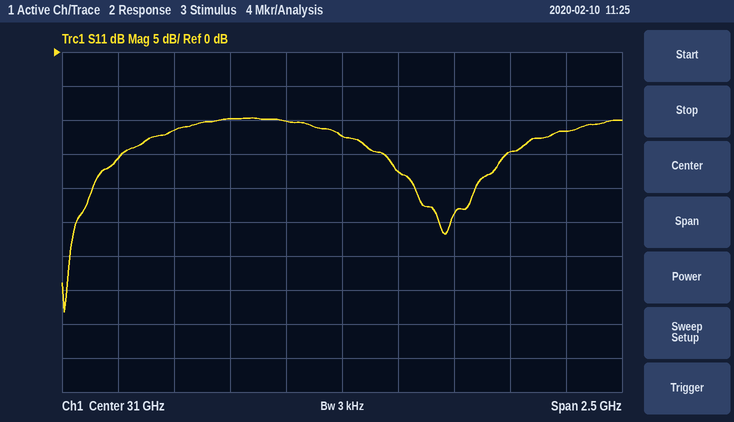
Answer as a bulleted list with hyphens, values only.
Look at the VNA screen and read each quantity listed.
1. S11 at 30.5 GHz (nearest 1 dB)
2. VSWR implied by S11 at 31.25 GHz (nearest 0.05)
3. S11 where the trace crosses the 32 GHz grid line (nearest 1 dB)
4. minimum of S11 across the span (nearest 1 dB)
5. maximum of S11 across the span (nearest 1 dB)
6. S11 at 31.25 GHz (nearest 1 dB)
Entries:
- -10 dB
- 1.30
- -12 dB
- -38 dB
- -10 dB
- -18 dB
